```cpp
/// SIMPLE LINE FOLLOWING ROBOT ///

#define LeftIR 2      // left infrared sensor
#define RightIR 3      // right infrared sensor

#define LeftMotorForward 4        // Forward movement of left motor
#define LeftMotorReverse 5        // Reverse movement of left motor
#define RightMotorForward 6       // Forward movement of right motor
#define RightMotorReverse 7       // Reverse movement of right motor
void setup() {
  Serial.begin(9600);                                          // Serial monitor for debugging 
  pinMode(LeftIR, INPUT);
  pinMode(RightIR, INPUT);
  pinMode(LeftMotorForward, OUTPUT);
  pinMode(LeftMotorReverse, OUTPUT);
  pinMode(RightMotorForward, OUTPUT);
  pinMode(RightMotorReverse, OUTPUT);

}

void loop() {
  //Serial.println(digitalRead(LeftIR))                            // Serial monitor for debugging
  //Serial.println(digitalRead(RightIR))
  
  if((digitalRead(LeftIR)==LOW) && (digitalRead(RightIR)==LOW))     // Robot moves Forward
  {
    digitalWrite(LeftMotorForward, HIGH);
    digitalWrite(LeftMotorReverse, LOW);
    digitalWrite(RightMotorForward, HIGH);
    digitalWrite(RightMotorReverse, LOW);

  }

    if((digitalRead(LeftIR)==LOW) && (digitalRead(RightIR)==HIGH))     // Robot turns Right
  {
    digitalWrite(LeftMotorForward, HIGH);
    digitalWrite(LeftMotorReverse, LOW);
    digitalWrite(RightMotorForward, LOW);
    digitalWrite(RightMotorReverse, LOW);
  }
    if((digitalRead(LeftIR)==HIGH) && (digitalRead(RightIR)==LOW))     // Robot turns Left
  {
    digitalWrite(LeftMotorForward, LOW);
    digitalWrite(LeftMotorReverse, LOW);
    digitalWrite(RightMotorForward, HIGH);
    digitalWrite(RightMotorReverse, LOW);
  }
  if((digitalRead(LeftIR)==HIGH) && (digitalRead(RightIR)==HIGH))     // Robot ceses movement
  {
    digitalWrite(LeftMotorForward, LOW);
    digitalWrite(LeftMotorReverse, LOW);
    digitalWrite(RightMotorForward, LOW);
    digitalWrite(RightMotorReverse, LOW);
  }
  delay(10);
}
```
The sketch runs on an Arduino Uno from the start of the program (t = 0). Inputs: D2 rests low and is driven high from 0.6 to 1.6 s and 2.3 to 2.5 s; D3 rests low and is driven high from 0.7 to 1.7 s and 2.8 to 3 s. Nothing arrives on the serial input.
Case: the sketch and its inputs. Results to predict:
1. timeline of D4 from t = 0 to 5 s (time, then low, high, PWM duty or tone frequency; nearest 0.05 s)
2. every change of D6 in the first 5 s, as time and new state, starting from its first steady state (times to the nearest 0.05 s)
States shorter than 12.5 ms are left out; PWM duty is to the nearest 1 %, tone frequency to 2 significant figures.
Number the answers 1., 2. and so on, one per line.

1. 0 s high; 0.6 s low; 1.6 s high; 2.3 s low; 2.5 s high
2. 0 s high; 0.7 s low; 1.7 s high; 2.8 s low; 3 s high
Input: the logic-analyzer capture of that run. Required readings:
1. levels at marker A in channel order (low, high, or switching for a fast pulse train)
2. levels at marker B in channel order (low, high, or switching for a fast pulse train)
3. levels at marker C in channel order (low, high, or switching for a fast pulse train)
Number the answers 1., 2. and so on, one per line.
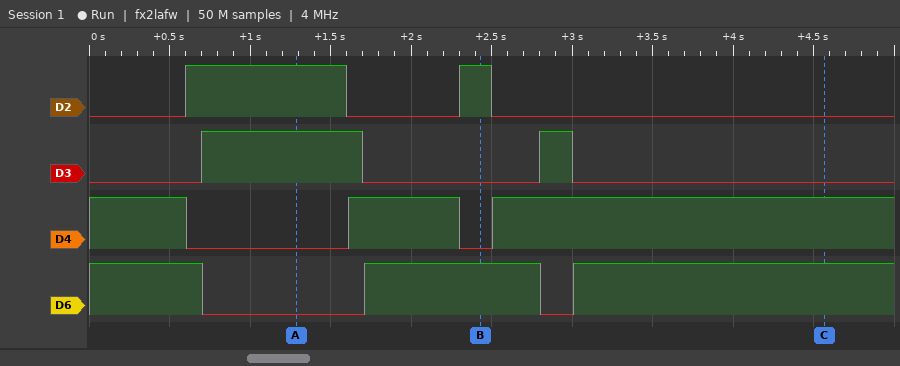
1. D2 high, D3 high, D4 low, D6 low
2. D2 high, D3 low, D4 low, D6 high
3. D2 low, D3 low, D4 high, D6 high
